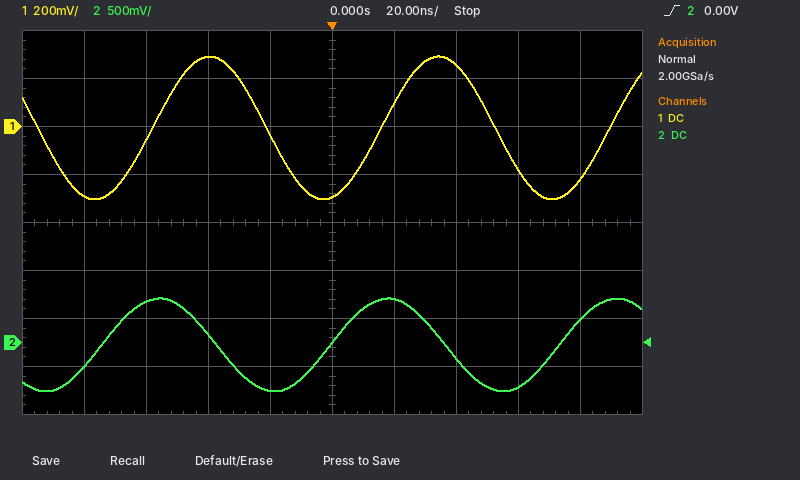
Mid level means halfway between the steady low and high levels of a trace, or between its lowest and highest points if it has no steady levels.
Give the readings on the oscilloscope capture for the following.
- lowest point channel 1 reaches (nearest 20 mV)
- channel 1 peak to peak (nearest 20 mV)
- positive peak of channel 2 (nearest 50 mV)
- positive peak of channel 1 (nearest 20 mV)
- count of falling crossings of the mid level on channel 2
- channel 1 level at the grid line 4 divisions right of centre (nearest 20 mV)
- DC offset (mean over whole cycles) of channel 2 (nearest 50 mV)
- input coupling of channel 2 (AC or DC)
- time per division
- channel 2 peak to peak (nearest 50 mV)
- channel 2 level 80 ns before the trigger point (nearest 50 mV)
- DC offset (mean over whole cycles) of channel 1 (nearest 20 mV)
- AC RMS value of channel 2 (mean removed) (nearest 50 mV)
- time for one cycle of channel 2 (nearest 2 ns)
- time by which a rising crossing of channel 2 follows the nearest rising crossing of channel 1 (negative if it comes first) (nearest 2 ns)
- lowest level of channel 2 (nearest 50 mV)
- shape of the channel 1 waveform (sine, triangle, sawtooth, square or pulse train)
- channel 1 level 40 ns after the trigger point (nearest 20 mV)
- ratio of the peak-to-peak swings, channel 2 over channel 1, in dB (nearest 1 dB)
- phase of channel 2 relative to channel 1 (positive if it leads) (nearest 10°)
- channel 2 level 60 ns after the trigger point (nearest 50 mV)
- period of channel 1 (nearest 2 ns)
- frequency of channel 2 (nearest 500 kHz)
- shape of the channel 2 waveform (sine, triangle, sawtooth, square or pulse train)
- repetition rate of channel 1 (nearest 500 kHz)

-300 mV
600 mV
450 mV
300 mV
2
-220 mV
0 mV
DC
20 ns
950 mV
-250 mV
0 mV
350 mV
74 ns
-16 ns
-500 mV
sine
260 mV
4 dB
+80°
-450 mV
74 ns
13.5 MHz
sine
13.5 MHz
